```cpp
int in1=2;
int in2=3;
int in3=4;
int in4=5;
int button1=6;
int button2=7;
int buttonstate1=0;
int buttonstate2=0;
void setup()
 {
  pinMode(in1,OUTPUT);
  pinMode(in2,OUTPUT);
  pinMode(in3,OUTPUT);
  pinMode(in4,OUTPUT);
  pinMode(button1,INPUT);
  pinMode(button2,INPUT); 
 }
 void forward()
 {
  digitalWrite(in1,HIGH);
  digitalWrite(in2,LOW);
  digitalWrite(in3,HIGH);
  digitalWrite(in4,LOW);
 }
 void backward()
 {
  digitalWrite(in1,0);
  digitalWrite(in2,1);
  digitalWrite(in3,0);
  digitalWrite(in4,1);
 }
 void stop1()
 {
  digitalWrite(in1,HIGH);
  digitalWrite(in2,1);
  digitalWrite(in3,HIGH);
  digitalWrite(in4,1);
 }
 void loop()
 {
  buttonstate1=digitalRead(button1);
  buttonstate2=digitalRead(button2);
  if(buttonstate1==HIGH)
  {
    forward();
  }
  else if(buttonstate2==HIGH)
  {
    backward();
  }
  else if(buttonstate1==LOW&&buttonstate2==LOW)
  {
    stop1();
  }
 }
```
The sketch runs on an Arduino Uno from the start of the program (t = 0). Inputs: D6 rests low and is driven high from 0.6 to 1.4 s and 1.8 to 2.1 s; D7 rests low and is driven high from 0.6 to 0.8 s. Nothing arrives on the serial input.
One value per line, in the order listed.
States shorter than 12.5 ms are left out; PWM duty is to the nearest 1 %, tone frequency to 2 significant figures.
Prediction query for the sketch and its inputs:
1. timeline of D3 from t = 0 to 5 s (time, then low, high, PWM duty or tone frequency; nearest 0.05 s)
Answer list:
0 s high; 0.6 s low; 1.4 s high; 1.8 s low; 2.1 s high
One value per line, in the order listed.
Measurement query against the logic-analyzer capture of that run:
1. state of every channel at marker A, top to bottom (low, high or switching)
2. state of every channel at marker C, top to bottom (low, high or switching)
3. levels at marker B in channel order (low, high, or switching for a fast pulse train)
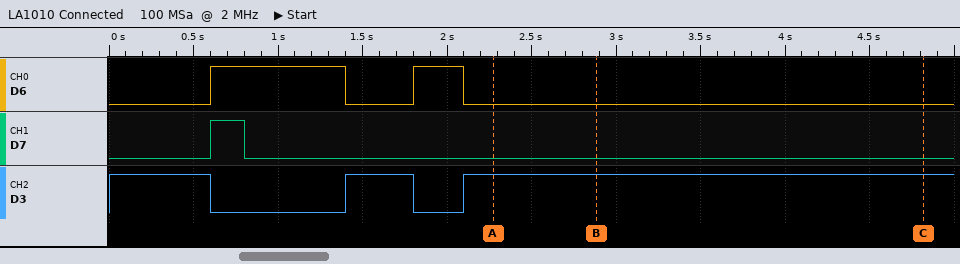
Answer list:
D6 low, D7 low, D3 high
D6 low, D7 low, D3 high
D6 low, D7 low, D3 high
